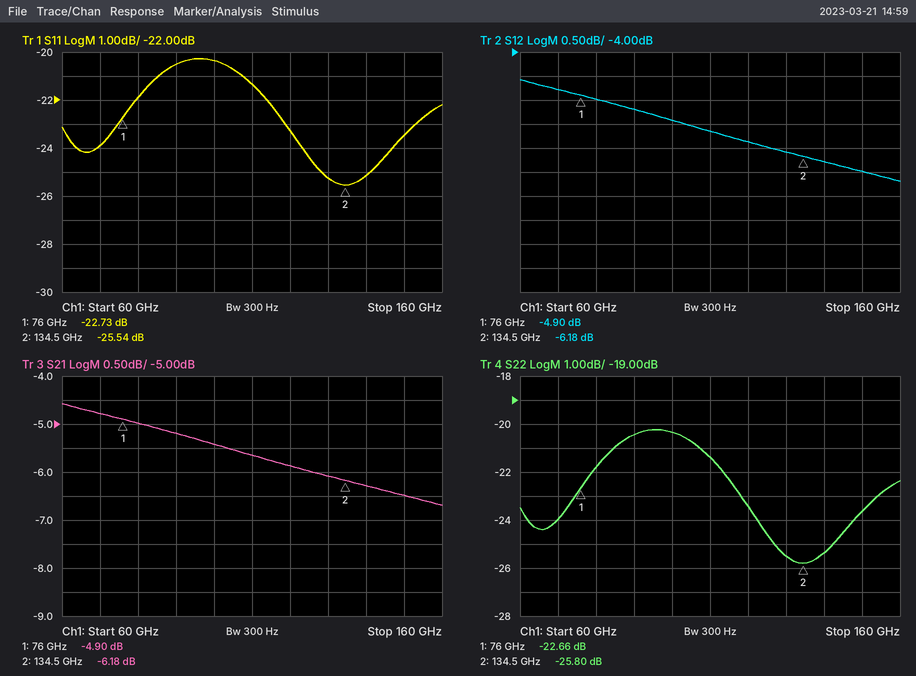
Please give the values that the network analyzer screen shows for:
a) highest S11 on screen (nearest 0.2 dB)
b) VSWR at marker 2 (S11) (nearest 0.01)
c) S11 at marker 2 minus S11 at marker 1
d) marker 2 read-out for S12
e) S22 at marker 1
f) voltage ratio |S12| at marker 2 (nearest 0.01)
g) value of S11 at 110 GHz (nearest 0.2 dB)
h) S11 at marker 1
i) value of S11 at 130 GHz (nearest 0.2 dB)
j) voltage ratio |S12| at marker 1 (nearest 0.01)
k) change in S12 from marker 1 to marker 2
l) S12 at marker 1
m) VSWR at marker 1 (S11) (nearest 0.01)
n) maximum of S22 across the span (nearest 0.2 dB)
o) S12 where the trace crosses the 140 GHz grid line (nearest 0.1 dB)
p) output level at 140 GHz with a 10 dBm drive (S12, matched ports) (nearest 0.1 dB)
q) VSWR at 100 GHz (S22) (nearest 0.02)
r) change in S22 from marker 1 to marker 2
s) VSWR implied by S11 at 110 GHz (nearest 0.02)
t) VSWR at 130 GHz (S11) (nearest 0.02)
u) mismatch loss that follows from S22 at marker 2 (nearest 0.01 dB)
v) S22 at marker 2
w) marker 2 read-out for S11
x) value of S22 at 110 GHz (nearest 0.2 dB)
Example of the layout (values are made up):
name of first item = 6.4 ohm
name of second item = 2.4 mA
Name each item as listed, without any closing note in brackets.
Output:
highest S11 on screen = -20.2 dB
VSWR at marker 2 (S11) = 1.11
S11 at marker 2 minus S11 at marker 1 = -2.81 dB
marker 2 read-out for S12 = -6.18 dB
S22 at marker 1 = -22.66 dB
voltage ratio |S12| at marker 2 = 0.49
value of S11 at 110 GHz = -21.4 dB
S11 at marker 1 = -22.73 dB
value of S11 at 130 GHz = -25.2 dB
voltage ratio |S12| at marker 1 = 0.57
change in S12 from marker 1 to marker 2 = -1.28 dB
S12 at marker 1 = -4.90 dB
VSWR at marker 1 (S11) = 1.16
maximum of S22 across the span = -20.2 dB
S12 where the trace crosses the 140 GHz grid line = -6.3 dB
output level at 140 GHz with a 10 dBm drive (S12, matched ports) = 3.7 dBm
VSWR at 100 GHz (S22) = 1.22
change in S22 from marker 1 to marker 2 = -3.14 dB
VSWR implied by S11 at 110 GHz = 1.18
VSWR at 130 GHz (S11) = 1.12
mismatch loss that follows from S22 at marker 2 = 0.01 dB
S22 at marker 2 = -25.80 dB
marker 2 read-out for S11 = -25.54 dB
value of S22 at 110 GHz = -21.4 dB
